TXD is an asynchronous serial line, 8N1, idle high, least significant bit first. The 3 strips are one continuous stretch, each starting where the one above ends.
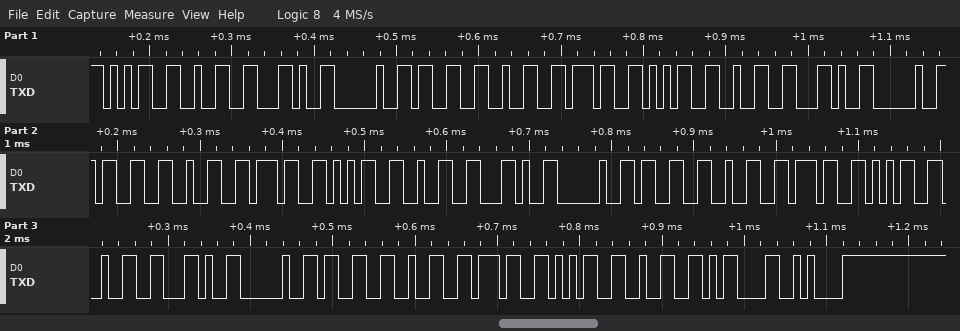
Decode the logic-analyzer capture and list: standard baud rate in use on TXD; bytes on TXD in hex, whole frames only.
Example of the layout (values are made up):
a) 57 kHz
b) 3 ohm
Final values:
a) 115200 baud
b) 0x35 0x32 0x2C 0x20 0x33 0x32 0x37 0x35 0x32 0x2C 0x20 0x33 0x32 0x37 0x35 0x32 0x2C 0x20 0x33 0x32 0x37 0x35 0x32 0x2C 0x20 0x33 0x32 0x37 0x35 0x32 0x0D 0x0A
